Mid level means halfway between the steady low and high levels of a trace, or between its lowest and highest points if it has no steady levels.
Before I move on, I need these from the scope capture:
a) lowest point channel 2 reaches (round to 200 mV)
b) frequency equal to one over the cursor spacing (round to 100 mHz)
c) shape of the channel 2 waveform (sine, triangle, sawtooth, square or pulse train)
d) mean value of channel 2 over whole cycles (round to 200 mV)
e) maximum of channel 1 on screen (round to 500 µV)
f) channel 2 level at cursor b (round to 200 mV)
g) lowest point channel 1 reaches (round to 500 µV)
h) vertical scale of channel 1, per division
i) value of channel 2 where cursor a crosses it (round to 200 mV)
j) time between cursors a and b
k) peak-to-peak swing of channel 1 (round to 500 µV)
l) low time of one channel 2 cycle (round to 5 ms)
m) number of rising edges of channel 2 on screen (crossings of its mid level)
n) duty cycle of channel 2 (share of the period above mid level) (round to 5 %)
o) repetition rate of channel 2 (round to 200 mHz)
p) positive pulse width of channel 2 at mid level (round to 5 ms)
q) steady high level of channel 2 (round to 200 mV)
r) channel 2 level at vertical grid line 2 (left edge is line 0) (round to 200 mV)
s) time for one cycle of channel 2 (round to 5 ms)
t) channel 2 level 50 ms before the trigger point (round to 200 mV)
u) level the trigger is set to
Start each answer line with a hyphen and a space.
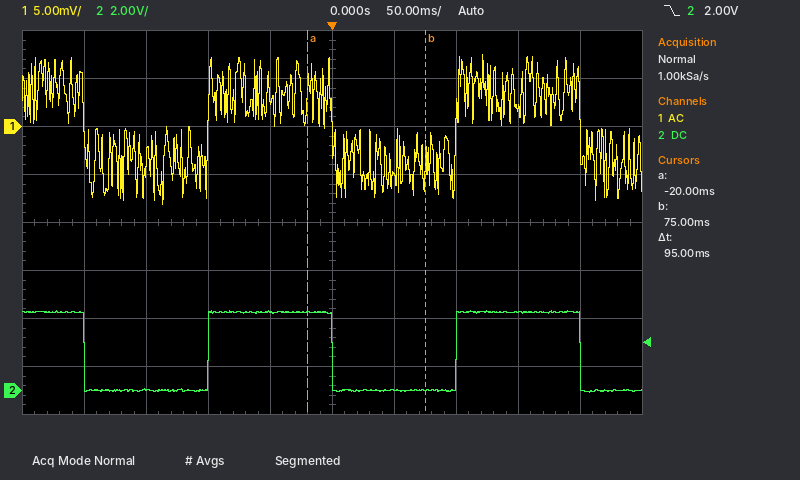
- 0.0 V
- 10.5 Hz
- square
- 1.6 V
- 7.5 mV
- 0.0 V
- -8.0 mV
- 5 mV
- 3.2 V
- 95 ms
- 15.5 mV
- 100 ms
- 2
- 50 %
- 5.0 Hz
- 100 ms
- 3.2 V
- 0.0 V
- 200 ms
- 3.2 V
- 2.00 V
